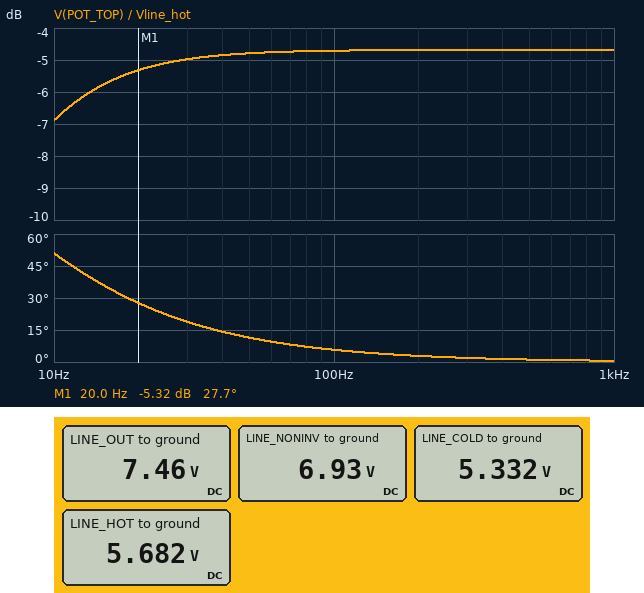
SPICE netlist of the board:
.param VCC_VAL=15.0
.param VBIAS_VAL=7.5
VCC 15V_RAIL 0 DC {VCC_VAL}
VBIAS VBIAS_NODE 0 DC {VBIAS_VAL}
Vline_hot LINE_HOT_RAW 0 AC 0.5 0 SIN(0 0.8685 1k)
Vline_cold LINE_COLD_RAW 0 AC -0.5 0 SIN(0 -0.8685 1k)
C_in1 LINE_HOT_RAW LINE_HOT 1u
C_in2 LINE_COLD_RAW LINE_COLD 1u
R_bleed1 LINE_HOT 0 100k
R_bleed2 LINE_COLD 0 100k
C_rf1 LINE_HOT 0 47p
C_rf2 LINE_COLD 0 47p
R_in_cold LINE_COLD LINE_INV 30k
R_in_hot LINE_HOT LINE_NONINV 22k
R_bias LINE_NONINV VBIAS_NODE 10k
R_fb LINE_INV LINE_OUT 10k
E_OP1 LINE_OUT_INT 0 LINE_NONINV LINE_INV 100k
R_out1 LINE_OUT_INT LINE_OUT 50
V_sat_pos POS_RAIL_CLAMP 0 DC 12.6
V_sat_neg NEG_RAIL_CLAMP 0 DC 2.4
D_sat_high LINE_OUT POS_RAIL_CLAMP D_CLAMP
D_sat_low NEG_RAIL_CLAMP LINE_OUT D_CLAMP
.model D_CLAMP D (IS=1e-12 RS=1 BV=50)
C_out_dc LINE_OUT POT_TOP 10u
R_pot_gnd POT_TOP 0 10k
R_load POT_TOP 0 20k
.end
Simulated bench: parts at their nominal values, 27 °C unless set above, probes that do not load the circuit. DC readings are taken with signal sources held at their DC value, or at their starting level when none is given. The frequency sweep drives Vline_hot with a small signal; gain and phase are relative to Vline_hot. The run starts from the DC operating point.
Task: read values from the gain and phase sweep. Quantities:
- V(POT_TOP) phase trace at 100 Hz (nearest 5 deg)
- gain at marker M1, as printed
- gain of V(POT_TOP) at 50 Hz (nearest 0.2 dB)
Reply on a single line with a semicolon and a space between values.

5 deg; -5.32 dB; -4.8 dB
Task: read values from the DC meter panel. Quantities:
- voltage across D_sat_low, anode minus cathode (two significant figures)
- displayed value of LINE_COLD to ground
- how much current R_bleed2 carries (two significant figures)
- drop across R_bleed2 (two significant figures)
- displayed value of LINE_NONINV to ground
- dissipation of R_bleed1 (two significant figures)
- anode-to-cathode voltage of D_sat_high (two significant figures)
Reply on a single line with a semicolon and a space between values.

-5.1 V; 5.332 V; 53 µA; 5.3 V; 6.93 V; 320 µW; -5.1 V
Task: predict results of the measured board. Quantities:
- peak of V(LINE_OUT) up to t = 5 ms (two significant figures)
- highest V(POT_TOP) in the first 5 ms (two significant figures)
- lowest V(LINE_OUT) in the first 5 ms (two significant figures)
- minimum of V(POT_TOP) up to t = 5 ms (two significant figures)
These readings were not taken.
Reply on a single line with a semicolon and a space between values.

8.1 V; 650 mV; 6.8 V; -660 mV
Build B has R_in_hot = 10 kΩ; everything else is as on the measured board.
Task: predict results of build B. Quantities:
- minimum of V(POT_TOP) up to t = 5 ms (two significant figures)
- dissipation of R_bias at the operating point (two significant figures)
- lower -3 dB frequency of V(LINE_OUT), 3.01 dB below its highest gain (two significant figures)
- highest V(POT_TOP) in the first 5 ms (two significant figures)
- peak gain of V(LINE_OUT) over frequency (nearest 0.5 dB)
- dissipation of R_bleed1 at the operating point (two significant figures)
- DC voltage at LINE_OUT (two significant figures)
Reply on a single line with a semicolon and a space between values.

-880 mV; 39 µW; 10 Hz; 860 mV; -1.5 dB; 390 µW; 7.4 V
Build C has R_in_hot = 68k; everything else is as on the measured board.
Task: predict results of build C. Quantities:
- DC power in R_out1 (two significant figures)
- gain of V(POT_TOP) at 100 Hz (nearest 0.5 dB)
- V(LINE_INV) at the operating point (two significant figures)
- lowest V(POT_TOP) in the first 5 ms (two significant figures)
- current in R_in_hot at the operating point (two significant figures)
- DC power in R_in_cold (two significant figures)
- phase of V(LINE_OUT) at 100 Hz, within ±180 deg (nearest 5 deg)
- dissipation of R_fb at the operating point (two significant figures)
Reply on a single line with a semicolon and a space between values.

150 nW; -9.5 dB; 7.1 V; -440 mV; 42 µA; 89 µW; 5 deg; 30 µW
